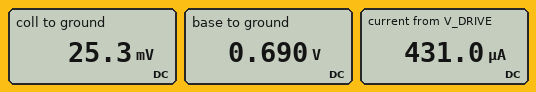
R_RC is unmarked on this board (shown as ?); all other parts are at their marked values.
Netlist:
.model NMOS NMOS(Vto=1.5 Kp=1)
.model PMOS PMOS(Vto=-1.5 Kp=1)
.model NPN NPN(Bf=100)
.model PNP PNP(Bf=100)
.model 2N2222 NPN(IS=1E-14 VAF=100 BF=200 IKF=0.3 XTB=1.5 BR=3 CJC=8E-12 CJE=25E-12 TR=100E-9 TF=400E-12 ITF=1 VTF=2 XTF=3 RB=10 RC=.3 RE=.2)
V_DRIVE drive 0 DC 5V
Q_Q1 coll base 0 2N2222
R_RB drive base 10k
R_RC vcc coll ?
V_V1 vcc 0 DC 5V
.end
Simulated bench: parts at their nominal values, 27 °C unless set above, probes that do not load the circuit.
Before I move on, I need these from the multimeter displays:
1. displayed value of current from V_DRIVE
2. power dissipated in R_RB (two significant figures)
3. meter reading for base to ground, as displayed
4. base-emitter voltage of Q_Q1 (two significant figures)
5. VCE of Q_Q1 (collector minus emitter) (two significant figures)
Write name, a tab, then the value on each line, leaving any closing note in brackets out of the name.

displayed value of current from V_DRIVE	431.0 µA
power dissipated in R_RB	1.9 mW
meter reading for base to ground, as displayed	0.690 V
base-emitter voltage of Q_Q1	690 mV
VCE of Q_Q1 (collector minus emitter)	25 mV
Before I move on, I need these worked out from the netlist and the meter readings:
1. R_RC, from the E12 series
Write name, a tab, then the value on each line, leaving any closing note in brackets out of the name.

R_RC, from the E12 series	3.3 kΩ
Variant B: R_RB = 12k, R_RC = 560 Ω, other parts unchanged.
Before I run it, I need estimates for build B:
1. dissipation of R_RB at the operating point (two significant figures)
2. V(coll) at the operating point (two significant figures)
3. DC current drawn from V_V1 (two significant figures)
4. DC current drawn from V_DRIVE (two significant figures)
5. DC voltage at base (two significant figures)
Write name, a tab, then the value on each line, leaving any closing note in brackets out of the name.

dissipation of R_RB at the operating point	1.5 mW
V(coll) at the operating point	67 mV
DC current drawn from V_V1	8.8 mA
DC current drawn from V_DRIVE	360 µA
DC voltage at base	720 mV
